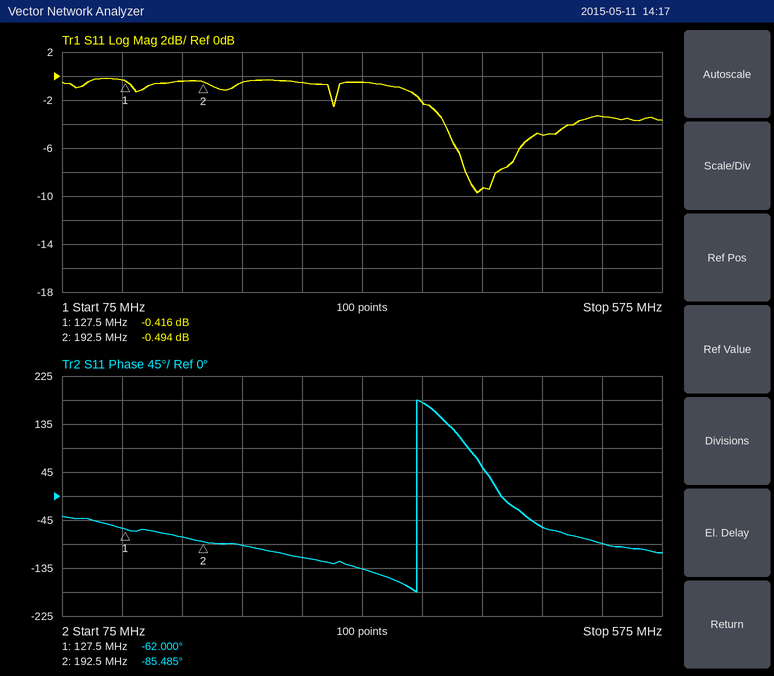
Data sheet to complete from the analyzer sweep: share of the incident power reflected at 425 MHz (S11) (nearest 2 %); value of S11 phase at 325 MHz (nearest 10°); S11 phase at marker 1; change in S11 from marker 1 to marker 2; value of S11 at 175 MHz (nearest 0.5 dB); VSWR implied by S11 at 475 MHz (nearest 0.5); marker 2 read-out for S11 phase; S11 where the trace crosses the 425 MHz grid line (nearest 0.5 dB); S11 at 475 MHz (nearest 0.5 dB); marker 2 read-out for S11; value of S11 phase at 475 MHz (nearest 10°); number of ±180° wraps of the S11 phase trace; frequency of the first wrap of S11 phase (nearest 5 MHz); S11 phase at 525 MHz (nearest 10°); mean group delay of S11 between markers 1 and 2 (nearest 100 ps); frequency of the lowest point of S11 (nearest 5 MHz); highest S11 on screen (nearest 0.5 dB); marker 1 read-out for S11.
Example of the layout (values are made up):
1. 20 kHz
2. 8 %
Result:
1. 12 %
2. -140°
3. -62.000°
4. -0.078 dB
5. -0.5 dB
6. 3.5
7. -85.485°
8. -9.5 dB
9. -5.0 dB
10. -0.494 dB
11. -60°
12. 1
13. 370 MHz
14. -90°
15. 1.0 ns
16. 420 MHz
17. 0.0 dB
18. -0.416 dB
